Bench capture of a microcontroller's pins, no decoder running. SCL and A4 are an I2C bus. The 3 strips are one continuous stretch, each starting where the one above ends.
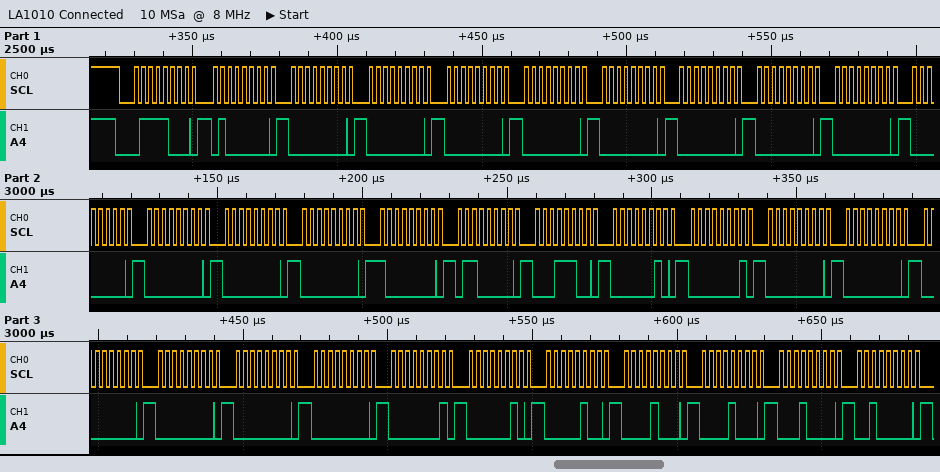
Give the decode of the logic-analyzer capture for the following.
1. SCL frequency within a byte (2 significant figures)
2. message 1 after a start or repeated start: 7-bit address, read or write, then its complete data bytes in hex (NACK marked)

400 kHz
0x3C write: 40 00 00 00 00 00 00 00 00 00 00 00 00 80 60 1C 02 01 00 00 00 00 00 00 01 02 04 08 08 10 20
